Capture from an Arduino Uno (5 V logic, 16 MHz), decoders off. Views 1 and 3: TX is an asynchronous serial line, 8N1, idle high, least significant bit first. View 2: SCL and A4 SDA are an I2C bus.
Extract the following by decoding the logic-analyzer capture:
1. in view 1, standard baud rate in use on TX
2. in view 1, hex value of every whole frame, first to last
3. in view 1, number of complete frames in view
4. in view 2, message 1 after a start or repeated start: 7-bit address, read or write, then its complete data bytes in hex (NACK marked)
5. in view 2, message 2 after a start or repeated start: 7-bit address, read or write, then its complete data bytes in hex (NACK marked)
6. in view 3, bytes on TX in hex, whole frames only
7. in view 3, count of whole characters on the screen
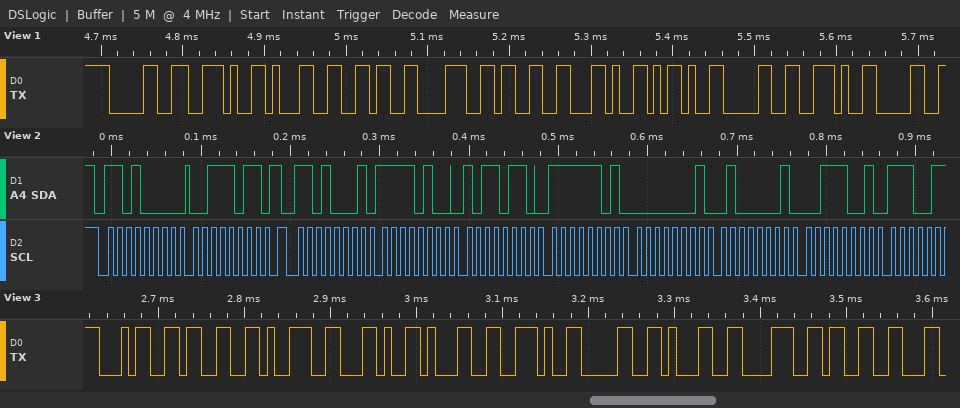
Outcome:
115200 baud
0x30 0x2E 0x31 0x36 0x38 0x33 0x2C 0x2D 0x30 0x2E 0x30
11
0x68 write: 3B
0x68 read: F4 B6 FD 01 41 39
0x34 0x33 0x39 0x2C 0x31 0x2E 0x30 0x31 0x38 0x33
10
